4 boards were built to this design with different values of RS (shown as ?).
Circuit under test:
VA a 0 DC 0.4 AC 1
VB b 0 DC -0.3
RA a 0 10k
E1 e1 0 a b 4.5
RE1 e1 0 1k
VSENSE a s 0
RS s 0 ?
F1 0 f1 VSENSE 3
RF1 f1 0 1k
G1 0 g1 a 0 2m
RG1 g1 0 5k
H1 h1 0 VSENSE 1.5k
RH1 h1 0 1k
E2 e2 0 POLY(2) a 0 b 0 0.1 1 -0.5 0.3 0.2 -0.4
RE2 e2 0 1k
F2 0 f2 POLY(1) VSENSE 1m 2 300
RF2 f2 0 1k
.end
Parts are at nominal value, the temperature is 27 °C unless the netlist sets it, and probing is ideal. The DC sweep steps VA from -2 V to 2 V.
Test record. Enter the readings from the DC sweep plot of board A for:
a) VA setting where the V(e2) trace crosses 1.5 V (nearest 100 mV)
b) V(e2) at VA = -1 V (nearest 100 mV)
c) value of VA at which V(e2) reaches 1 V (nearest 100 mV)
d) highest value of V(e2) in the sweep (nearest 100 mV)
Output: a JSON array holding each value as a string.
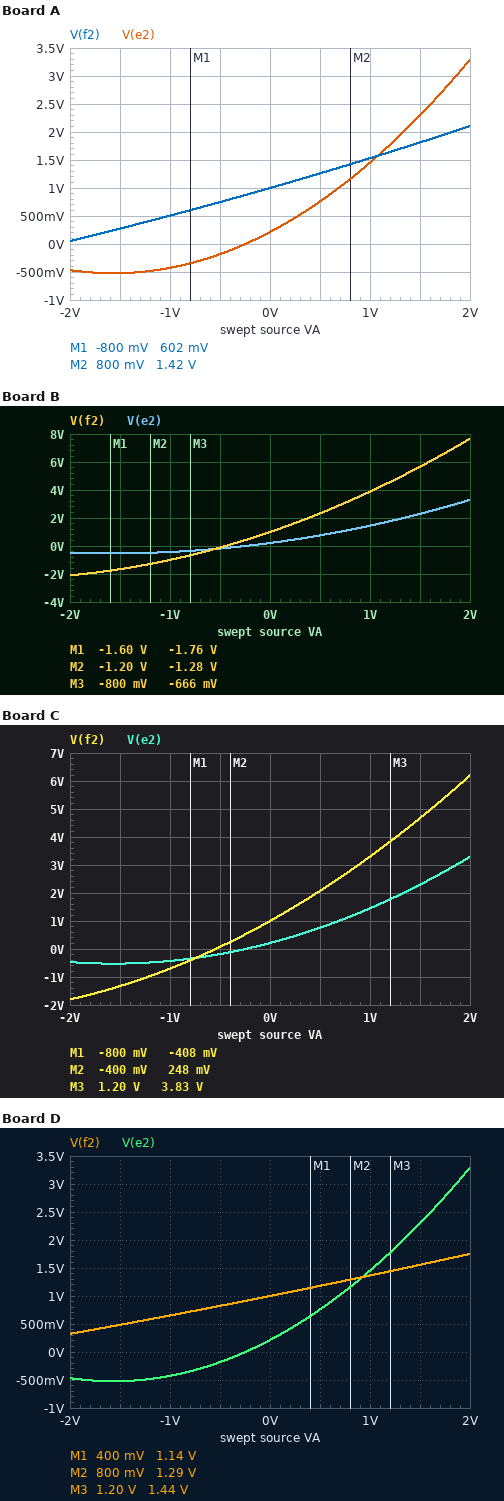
["1.0 V", "-400 mV", "700 mV", "3.3 V"]
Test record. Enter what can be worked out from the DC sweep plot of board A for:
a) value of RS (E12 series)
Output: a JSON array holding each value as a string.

["3.9 kΩ"]
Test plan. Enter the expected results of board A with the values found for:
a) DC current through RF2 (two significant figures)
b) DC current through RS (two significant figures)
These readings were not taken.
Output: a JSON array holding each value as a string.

["1.2 mA", "100 µA"]
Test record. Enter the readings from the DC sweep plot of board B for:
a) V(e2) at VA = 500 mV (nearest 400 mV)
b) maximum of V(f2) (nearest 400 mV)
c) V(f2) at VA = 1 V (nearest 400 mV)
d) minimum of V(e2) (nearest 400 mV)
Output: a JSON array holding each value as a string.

["800 mV", "7.6 V", "4.0 V", "-400 mV"]
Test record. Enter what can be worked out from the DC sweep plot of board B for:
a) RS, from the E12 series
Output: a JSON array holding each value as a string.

["820 Ω"]
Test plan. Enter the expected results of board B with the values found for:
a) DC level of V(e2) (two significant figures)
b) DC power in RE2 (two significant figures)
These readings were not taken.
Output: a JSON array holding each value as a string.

["640 mV", "410 µW"]
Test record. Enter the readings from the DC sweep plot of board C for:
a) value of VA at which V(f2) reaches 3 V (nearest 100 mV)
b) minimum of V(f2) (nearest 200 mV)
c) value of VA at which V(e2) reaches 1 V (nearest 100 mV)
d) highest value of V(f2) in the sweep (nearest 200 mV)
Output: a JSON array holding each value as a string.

["900 mV", "-1.8 V", "700 mV", "6.2 V"]
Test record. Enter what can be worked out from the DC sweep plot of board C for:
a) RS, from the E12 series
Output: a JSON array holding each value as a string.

["1 kΩ"]
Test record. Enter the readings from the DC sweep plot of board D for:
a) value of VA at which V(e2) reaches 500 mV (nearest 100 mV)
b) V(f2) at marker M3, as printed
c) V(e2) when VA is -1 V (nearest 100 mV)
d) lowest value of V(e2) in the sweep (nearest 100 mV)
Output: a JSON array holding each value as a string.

["300 mV", "1.44 V", "-400 mV", "-500 mV"]
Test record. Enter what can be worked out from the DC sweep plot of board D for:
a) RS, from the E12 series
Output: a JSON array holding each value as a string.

["5.6 kΩ"]
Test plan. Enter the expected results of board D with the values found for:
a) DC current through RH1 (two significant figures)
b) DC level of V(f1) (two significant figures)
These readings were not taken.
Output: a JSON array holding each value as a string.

["110 µA", "210 mV"]
